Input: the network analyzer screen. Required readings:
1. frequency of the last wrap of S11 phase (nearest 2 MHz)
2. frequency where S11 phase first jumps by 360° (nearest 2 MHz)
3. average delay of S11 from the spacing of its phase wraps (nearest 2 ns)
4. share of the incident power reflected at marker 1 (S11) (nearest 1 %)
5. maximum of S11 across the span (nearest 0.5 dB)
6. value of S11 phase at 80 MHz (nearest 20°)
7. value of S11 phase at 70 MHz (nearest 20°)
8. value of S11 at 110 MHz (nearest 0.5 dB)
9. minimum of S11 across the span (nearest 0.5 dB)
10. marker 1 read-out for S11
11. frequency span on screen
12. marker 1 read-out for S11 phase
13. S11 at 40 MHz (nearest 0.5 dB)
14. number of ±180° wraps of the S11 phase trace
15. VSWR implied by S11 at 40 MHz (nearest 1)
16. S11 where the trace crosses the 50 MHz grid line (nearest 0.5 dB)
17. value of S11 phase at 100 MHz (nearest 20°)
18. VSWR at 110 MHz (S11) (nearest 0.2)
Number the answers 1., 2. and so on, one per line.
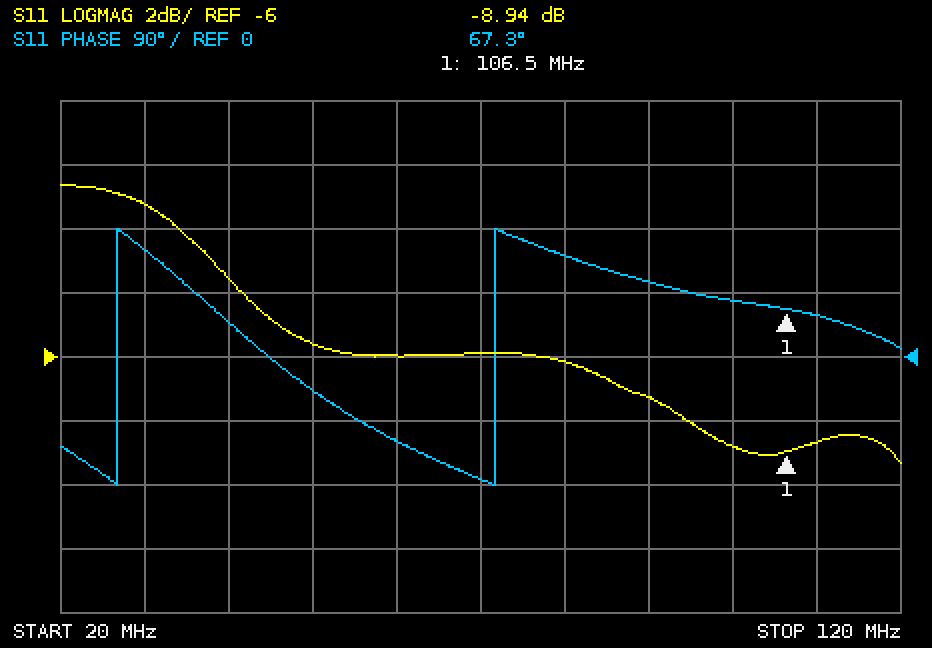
1. 72 MHz
2. 26 MHz
3. 22 ns
4. 13 %
5. -0.5 dB
6. 140°
7. -180°
8. -8.5 dB
9. -9.5 dB
10. -8.94 dB
11. 100 MHz
12. 67.3°
13. -3.5 dB
14. 2
15. 5
16. -5.5 dB
17. 80°
18. 2.2
